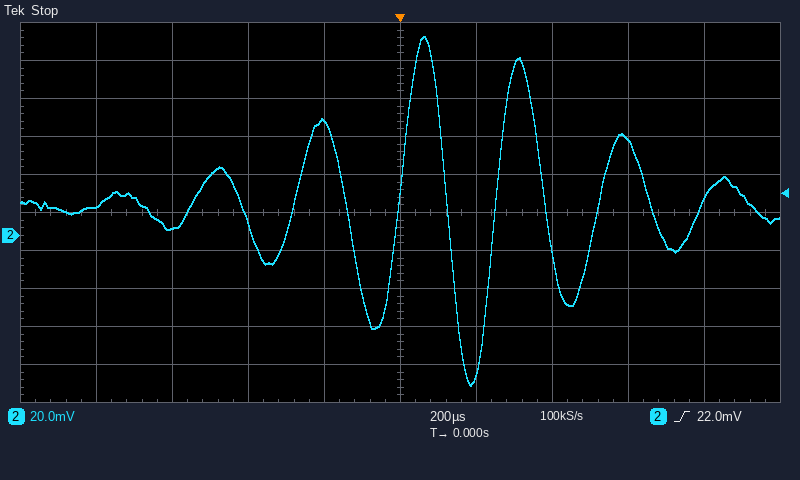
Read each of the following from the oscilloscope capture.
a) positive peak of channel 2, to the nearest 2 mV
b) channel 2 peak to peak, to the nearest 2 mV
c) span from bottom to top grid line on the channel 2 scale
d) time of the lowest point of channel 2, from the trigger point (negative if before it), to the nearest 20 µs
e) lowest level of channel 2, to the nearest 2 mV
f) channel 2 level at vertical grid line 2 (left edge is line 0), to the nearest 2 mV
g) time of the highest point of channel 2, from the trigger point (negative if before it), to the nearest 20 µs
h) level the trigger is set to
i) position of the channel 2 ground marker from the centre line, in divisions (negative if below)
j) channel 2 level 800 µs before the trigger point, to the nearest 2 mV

104 mV
184 mV
200 mV
+180 µs
-80 mV
4 mV
+60 µs
22.0 mV
-0.6 div
16 mV
